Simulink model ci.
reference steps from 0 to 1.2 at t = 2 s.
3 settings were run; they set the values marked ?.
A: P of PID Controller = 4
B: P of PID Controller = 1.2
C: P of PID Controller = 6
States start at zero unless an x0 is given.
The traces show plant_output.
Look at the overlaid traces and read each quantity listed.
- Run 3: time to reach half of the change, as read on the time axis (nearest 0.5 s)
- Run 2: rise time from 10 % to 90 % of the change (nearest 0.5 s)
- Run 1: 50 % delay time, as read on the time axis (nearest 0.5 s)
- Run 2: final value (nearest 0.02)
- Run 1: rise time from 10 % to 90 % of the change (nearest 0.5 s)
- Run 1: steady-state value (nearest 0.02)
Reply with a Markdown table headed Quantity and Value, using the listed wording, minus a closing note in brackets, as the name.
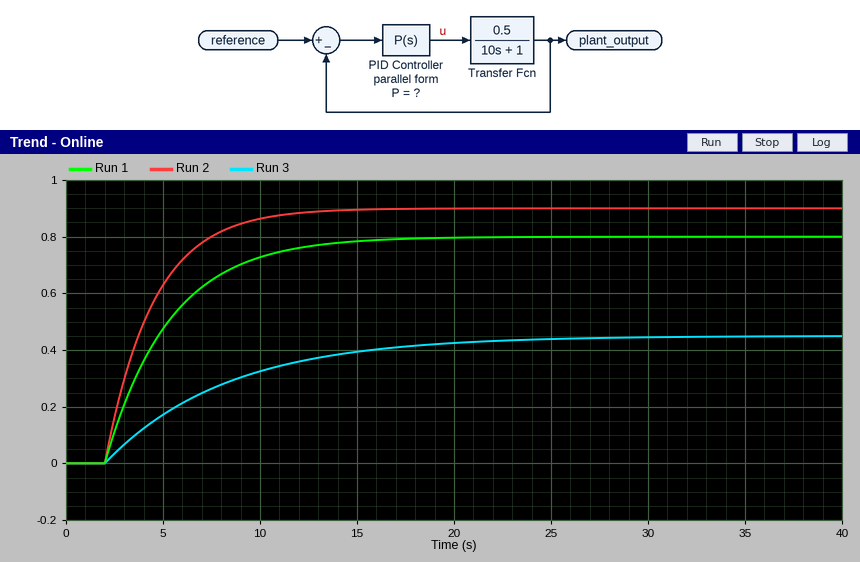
| Quantity | Value |
|---|---|
| Run 3: time to reach half of the change, as read on the time axis | 6.5 s |
| Run 2: rise time from 10 % to 90 % of the change | 5.5 s |
| Run 1: 50 % delay time, as read on the time axis | 4.5 s |
| Run 2: final value | 0.90 |
| Run 1: rise time from 10 % to 90 % of the change | 7.5 s |
| Run 1: steady-state value | 0.80 |
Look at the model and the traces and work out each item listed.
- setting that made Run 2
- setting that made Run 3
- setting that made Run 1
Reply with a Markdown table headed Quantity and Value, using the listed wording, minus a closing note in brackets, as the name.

| Quantity | Value |
|---|---|
| setting that made Run 2 | C |
| setting that made Run 3 | B |
| setting that made Run 1 | A |
